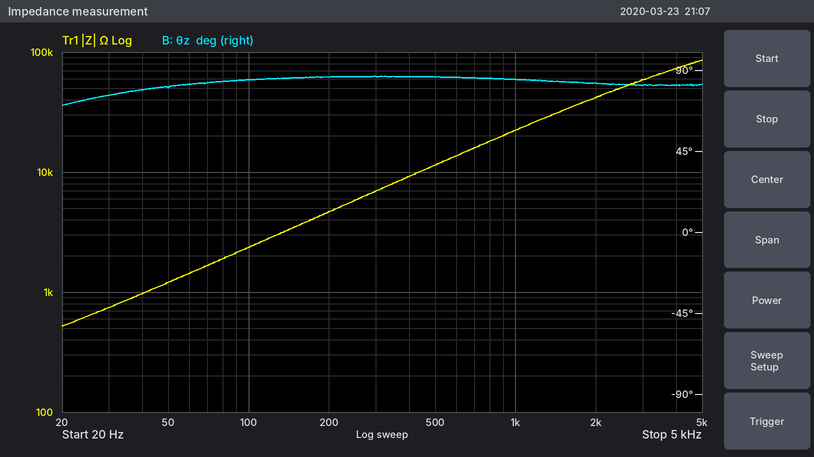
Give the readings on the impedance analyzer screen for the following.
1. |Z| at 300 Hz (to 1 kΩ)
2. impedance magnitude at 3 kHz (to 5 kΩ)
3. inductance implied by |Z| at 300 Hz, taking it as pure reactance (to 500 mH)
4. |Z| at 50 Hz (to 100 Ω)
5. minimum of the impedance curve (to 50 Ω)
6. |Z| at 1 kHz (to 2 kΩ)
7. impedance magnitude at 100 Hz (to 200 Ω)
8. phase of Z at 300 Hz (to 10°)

7 kΩ
60 kΩ
3.5 H
1.2 kΩ
500 Ω
22 kΩ
2.4 kΩ
90°
